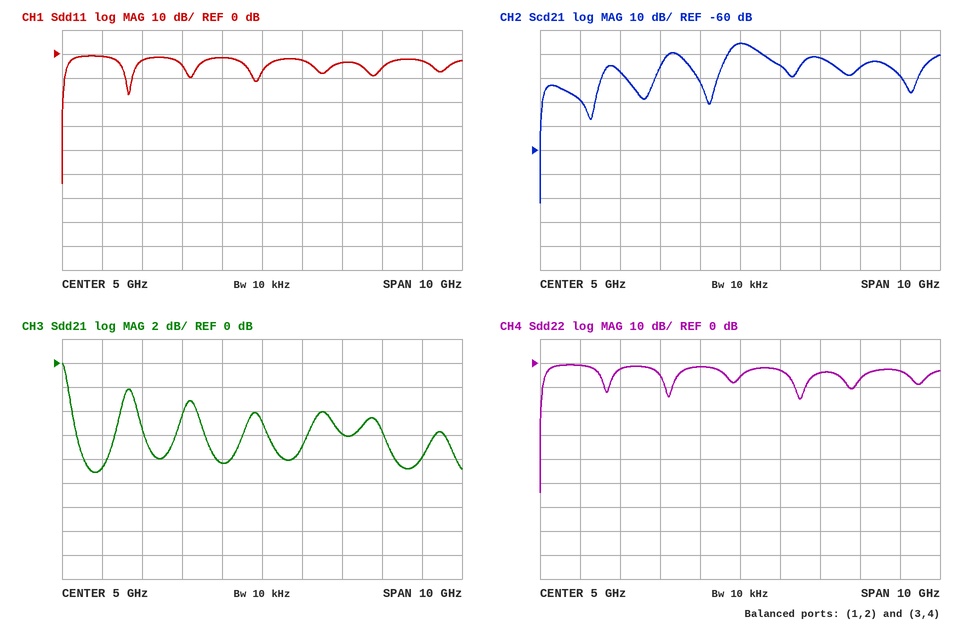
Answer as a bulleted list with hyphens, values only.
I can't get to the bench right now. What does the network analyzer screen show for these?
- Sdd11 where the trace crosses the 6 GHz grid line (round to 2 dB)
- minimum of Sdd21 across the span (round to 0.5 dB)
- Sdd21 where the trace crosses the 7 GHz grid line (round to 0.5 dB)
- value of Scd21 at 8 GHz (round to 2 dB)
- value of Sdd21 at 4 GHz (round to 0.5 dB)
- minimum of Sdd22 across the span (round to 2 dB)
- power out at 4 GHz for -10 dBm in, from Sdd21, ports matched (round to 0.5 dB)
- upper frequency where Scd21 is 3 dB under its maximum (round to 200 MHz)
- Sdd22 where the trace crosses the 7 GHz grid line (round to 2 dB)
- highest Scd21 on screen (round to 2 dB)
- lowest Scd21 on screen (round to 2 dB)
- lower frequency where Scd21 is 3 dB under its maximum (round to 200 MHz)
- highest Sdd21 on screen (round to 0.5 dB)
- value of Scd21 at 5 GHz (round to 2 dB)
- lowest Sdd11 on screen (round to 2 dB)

- -2 dB
- -9.0 dB
- -6.0 dB
- -26 dB
- -8.5 dB
- -54 dB
- -18.5 dBm
- 5.4 GHz
- -4 dB
- -16 dB
- -82 dB
- 4.8 GHz
- 0.0 dB
- -16 dB
- -54 dB
